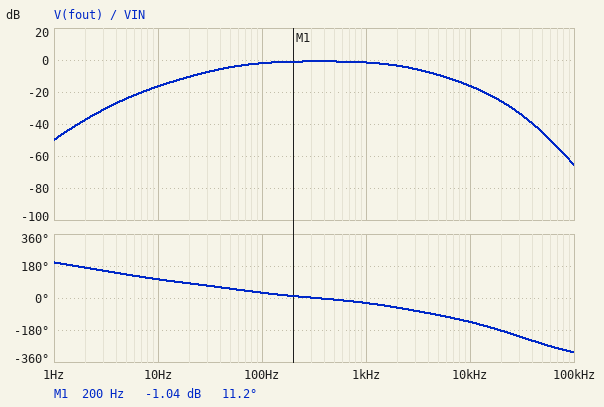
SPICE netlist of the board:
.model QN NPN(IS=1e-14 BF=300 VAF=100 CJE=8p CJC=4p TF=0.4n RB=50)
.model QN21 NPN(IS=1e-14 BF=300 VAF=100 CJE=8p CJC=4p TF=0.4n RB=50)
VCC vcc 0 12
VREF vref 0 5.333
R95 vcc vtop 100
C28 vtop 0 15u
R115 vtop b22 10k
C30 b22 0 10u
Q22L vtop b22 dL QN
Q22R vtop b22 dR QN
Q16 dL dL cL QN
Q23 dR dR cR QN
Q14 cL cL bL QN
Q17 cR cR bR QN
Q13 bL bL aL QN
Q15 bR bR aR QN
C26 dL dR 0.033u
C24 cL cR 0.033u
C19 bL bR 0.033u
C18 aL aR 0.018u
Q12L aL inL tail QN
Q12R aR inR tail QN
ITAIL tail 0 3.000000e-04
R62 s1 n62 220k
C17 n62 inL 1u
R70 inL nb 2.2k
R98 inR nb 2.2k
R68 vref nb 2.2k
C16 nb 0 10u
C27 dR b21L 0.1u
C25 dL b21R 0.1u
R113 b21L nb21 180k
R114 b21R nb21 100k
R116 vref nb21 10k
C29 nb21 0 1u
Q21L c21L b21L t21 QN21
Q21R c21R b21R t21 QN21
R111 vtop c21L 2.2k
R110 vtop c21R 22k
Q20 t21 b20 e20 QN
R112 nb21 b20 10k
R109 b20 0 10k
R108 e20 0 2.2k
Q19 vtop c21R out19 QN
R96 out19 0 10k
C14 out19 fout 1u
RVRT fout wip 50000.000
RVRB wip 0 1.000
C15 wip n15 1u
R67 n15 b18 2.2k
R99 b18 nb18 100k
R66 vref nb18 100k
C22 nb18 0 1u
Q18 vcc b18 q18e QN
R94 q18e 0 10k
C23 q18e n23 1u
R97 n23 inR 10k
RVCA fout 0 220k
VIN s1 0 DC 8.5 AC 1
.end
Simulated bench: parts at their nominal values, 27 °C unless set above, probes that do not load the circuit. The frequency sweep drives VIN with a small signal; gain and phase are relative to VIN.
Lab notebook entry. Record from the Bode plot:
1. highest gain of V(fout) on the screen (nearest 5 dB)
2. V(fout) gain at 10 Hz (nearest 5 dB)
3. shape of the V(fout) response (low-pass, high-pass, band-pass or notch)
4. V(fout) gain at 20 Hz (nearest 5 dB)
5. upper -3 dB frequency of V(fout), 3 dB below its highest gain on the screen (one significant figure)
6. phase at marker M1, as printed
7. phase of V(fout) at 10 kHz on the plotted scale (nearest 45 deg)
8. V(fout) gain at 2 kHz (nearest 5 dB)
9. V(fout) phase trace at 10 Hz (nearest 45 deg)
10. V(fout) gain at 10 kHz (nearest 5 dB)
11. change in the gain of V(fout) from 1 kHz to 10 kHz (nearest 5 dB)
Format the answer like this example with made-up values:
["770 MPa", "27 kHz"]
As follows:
["0 dB", "-15 dB", "band-pass", "-10 dB", "2 kHz", "11.2 deg", "-135 deg", "-5 dB", "90 deg", "-15 dB", "-15 dB"]
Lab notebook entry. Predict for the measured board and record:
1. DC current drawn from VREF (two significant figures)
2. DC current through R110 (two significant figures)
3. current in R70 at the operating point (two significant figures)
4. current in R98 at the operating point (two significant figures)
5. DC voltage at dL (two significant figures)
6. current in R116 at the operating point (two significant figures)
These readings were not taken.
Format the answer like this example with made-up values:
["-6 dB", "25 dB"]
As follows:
["180 µA", "310 µA", "480 nA", "480 nA", "11 V", "180 µA"]
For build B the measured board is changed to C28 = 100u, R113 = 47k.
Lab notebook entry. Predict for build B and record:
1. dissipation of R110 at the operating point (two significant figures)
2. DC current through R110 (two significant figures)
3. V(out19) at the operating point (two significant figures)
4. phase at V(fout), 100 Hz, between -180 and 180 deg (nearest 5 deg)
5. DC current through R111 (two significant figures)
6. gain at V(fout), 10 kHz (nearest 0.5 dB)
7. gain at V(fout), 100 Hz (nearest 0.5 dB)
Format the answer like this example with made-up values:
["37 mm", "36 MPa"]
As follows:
["790 µW", "190 µA", "7.0 V", "35 deg", "320 µA", "-16.5 dB", "-2.5 dB"]
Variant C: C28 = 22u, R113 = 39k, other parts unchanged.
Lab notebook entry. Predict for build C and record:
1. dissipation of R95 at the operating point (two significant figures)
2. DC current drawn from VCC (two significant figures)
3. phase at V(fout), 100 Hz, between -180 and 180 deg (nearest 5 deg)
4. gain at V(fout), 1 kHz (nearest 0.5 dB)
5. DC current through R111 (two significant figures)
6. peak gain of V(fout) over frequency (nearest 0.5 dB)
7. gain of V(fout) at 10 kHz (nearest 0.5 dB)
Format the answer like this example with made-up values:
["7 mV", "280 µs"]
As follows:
["240 µW", "2.0 mA", "35 deg", "-2.0 dB", "330 µA", "-1.5 dB", "-16.5 dB"]
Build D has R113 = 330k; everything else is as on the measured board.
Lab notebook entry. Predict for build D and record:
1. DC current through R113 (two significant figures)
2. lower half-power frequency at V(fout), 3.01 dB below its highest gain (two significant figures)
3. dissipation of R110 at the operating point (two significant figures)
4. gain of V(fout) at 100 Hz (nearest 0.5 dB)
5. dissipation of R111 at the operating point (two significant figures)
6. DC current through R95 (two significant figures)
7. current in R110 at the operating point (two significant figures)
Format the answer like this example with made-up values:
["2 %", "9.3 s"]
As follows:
["440 nA", "49 Hz", "2.9 mW", "-3.0 dB", "46 µW", "1.1 mA", "360 µA"]
